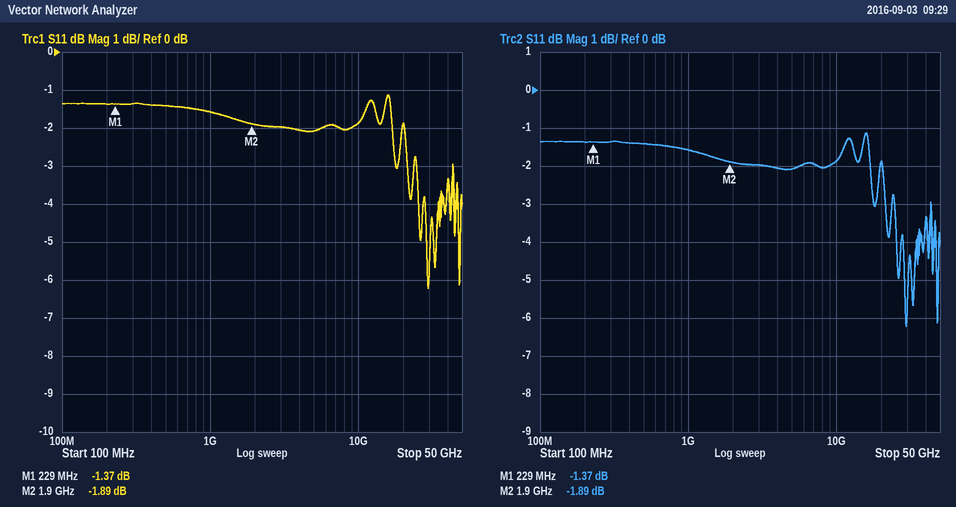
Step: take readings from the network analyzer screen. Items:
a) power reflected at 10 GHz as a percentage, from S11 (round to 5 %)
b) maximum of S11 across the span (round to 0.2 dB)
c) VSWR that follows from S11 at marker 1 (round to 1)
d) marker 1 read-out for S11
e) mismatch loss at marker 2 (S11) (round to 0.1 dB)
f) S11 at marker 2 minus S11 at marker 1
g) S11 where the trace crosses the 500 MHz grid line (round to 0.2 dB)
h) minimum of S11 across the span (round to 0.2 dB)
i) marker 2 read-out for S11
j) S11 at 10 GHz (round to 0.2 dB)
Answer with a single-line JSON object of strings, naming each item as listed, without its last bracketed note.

{"power reflected at 10 GHz as a percentage, from S11": "65 %", "maximum of S11 across the span": "-1.2 dB", "VSWR that follows from S11 at marker 1": "13", "marker 1 read-out for S11": "-1.37 dB", "mismatch loss at marker 2 (S11)": "4.5 dB", "S11 at marker 2 minus S11 at marker 1": "-0.52 dB", "S11 where the trace crosses the 500 MHz grid line": "-1.4 dB", "minimum of S11 across the span": "-6.2 dB", "marker 2 read-out for S11": "-1.89 dB", "S11 at 10 GHz": "-1.8 dB"}
